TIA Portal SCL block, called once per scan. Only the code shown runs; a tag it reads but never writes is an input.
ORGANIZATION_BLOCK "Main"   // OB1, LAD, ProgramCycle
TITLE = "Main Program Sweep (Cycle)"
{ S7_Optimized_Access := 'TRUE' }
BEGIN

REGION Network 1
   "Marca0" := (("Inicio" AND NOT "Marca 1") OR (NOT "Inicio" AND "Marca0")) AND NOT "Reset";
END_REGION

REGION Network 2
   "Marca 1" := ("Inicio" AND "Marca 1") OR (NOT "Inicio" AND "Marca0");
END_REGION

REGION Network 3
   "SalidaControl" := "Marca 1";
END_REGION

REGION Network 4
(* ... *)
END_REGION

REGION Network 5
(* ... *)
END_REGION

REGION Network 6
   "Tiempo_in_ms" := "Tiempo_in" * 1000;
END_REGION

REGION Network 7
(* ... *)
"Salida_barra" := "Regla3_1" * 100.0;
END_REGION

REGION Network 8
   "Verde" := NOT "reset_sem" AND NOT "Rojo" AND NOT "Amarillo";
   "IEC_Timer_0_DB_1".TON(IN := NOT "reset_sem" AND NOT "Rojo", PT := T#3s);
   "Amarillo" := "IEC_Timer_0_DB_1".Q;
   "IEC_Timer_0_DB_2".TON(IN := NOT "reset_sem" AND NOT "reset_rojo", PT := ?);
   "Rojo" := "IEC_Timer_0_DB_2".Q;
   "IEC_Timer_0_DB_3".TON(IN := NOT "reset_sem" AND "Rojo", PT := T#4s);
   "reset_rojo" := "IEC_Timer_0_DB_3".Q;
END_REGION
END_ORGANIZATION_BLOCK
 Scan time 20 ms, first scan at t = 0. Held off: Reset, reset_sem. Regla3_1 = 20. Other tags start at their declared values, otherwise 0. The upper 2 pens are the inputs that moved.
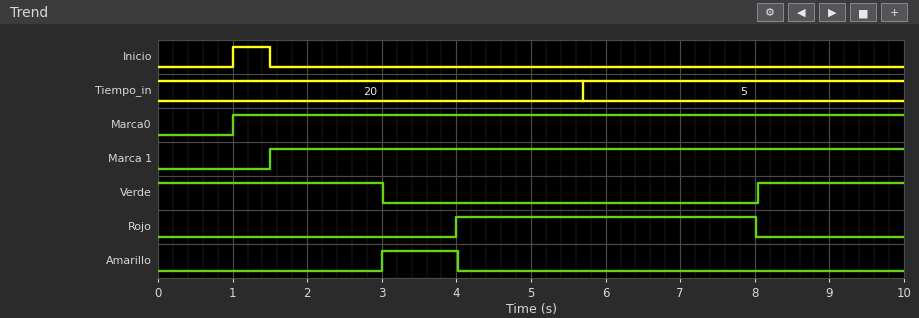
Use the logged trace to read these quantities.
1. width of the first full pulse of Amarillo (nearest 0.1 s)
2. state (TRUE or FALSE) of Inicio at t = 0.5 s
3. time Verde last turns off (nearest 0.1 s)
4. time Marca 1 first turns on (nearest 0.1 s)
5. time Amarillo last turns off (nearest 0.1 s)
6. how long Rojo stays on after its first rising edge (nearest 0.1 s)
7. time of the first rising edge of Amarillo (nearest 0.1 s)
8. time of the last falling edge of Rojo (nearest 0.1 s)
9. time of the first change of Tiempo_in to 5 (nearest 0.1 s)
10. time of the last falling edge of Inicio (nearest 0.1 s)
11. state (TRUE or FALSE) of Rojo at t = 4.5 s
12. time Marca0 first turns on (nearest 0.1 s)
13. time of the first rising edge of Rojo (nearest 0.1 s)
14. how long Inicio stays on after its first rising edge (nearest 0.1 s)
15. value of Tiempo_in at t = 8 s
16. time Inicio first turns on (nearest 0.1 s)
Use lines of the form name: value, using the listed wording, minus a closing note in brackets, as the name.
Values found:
width of the first full pulse of Amarillo: 1.0 s
state (TRUE or FALSE) of Inicio at t = 0.5 s: FALSE
time Verde last turns off: 3.0 s
time Marca 1 first turns on: 1.5 s
time Amarillo last turns off: 4.0 s
how long Rojo stays on after its first rising edge: 4.0 s
time of the first rising edge of Amarillo: 3.0 s
time of the last falling edge of Rojo: 8.0 s
time of the first change of Tiempo_in to 5: 5.7 s
time of the last falling edge of Inicio: 1.5 s
state (TRUE or FALSE) of Rojo at t = 4.5 s: TRUE
time Marca0 first turns on: 1.0 s
time of the first rising edge of Rojo: 4.0 s
how long Inicio stays on after its first rising edge: 0.5 s
value of Tiempo_in at t = 8 s: 5
time Inicio first turns on: 1.0 s
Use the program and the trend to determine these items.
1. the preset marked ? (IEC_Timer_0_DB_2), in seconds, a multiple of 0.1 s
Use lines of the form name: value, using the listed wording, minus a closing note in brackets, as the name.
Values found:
the preset marked ? (IEC_Timer_0_DB_2), in seconds, a multiple of 0.1 s: 4.0 s
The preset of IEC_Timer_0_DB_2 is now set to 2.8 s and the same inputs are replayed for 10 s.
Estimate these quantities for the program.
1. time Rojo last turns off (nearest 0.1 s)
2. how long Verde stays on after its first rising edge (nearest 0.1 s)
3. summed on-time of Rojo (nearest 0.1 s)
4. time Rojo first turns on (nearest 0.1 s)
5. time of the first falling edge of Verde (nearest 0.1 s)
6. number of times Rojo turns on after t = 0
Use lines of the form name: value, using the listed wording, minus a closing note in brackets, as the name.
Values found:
time Rojo last turns off: 6.8 s
how long Verde stays on after its first rising edge: 2.8 s
summed on-time of Rojo: 4.4 s
time Rojo first turns on: 2.8 s
time of the first falling edge of Verde: 2.8 s
number of times Rojo turns on after t = 0: 2
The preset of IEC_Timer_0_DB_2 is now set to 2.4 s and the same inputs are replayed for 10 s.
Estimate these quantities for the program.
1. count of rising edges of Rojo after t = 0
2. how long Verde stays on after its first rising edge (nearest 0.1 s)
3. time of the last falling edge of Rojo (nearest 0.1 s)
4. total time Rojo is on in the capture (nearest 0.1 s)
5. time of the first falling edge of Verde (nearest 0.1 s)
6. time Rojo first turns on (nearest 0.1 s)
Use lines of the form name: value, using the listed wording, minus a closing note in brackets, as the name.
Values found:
count of rising edges of Rojo after t = 0: 2
how long Verde stays on after its first rising edge: 2.4 s
time of the last falling edge of Rojo: 6.4 s
total time Rojo is on in the capture: 5.2 s
time of the first falling edge of Verde: 2.4 s
time Rojo first turns on: 2.4 s
